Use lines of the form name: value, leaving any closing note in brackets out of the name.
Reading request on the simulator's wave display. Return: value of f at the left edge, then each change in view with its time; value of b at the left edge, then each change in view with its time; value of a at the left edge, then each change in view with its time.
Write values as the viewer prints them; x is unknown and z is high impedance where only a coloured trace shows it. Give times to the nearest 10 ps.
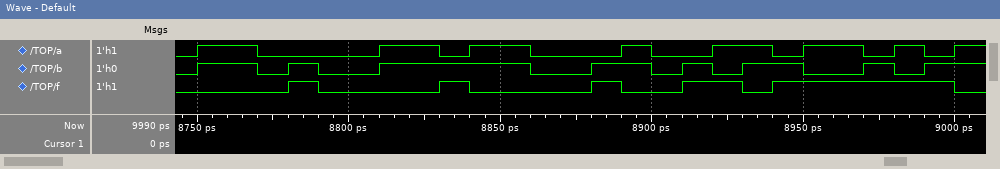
value of f at the left edge, then each change in view with its time: 0, 1 at 8780 ps, 0 at 8790 ps, 1 at 8830 ps, 0 at 8840 ps, 1 at 8880 ps, 0 at 8890 ps, 1 at 8910 ps, 0 at 8930 ps, 1 at 8940 ps, 0 at 9000 ps
value of b at the left edge, then each change in view with its time: 0, 1 at 8750 ps, 0 at 8770 ps, 1 at 8780 ps, 0 at 8790 ps, 1 at 8810 ps, 0 at 8860 ps, 1 at 8880 ps, 0 at 8900 ps, 1 at 8910 ps, 0 at 8920 ps, 1 at 8930 ps, 0 at 8950 ps, 1 at 8970 ps, 0 at 8980 ps, 1 at 8990 ps
value of a at the left edge, then each change in view with its time: 0, 1 at 8750 ps, 0 at 8770 ps, 1 at 8810 ps, 0 at 8830 ps, 1 at 8840 ps, 0 at 8860 ps, 1 at 8890 ps, 0 at 8900 ps, 1 at 8920 ps, 0 at 8940 ps, 1 at 8950 ps, 0 at 8970 ps, 1 at 8980 ps, 0 at 8990 ps, 1 at 9000 ps
